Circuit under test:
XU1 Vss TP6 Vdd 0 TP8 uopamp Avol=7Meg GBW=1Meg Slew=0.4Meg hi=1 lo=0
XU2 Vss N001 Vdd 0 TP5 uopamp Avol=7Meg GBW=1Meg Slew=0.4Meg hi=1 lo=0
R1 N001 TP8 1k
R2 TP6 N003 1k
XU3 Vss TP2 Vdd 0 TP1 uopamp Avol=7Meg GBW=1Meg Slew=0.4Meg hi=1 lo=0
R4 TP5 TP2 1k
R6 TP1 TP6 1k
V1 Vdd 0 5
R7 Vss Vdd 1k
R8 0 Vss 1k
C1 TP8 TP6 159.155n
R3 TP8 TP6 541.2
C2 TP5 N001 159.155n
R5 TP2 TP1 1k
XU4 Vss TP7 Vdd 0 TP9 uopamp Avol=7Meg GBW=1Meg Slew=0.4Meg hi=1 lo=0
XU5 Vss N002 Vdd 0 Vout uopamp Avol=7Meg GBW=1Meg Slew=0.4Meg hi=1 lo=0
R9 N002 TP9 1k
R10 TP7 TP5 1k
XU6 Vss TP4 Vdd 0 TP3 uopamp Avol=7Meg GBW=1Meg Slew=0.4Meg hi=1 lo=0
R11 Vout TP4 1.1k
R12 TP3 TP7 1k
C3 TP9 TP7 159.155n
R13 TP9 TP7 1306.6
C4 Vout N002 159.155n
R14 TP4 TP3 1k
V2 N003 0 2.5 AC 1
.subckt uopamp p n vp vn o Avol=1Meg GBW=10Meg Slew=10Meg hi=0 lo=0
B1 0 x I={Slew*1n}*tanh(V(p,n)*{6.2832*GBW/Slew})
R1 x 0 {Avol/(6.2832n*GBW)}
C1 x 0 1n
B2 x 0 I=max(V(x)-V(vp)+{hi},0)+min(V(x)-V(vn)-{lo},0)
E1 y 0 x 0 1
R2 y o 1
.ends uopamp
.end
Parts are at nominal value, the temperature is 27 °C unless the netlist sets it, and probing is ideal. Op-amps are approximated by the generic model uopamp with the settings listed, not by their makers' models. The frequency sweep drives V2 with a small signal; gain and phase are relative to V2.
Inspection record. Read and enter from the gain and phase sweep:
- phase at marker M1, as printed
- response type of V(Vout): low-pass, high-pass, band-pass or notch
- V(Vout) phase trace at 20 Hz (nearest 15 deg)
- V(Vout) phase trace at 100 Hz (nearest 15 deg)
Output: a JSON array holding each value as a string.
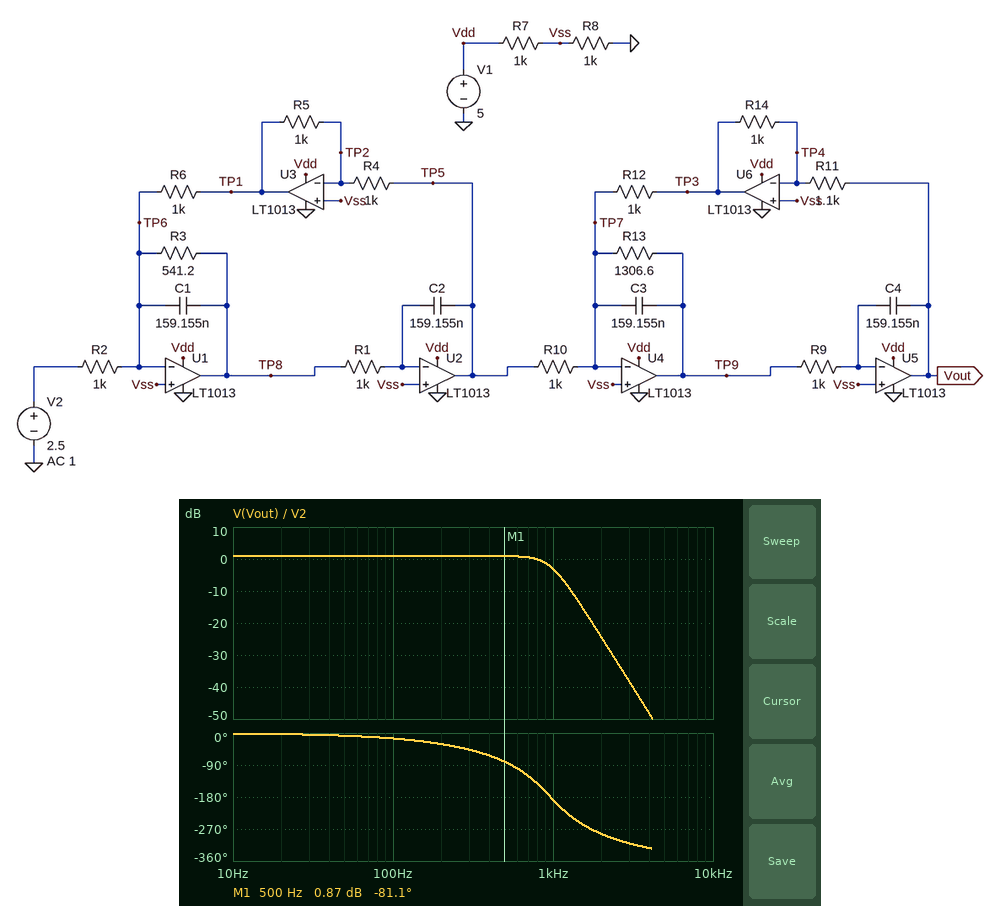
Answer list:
["-81.1 deg", "low-pass", "0 deg", "-15 deg"]
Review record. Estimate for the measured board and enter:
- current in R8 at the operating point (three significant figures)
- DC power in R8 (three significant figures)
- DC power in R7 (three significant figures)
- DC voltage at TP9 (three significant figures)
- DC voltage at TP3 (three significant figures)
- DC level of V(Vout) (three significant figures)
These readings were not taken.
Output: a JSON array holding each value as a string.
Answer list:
["2.50 mA", "6.25 mW", "6.25 mW", "2.50 V", "2.50 V", "2.50 V"]
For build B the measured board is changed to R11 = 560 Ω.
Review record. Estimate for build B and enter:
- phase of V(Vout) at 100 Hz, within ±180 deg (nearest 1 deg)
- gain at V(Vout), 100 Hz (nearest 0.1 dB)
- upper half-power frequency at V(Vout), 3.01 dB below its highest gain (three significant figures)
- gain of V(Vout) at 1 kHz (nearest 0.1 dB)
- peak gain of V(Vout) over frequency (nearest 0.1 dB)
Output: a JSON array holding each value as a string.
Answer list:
["-13 deg", "-5.1 dB", "1.31 kHz", "-6.1 dB", "-5.0 dB"]
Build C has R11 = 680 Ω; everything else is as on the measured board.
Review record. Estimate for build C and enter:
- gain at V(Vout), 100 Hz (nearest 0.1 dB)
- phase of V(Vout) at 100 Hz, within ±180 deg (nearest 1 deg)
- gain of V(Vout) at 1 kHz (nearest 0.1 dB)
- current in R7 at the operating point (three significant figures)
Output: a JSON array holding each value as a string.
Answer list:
["-3.4 dB", "-14 deg", "-4.3 dB", "2.50 mA"]
